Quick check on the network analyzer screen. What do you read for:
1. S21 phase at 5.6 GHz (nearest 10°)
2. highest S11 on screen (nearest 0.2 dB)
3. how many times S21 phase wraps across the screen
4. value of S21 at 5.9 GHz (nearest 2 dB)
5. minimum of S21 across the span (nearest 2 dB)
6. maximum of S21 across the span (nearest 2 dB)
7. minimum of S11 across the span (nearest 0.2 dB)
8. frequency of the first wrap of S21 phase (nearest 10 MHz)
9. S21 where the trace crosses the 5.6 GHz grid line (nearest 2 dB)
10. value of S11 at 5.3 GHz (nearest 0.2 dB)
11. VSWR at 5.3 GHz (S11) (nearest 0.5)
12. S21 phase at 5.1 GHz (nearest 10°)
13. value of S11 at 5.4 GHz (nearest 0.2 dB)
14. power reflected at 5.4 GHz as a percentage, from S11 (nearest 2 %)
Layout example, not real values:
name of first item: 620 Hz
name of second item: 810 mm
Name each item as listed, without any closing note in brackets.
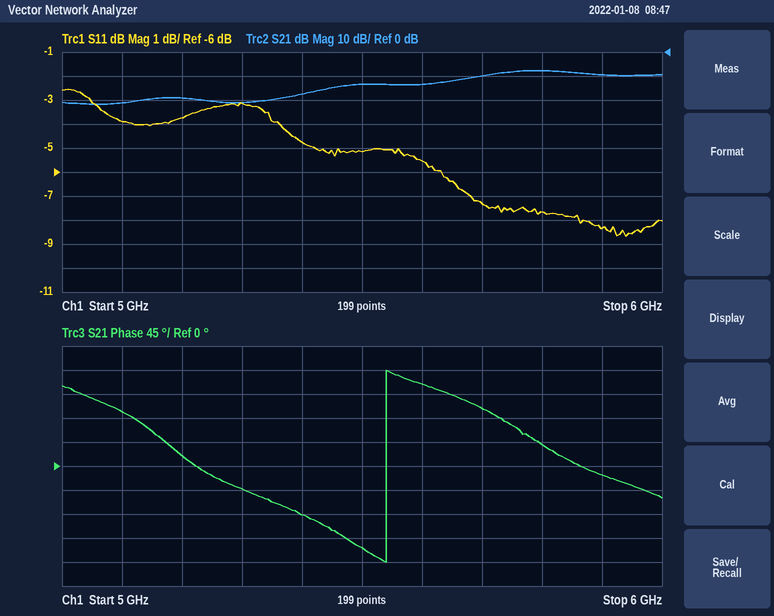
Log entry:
S21 phase at 5.6 GHz: 150°
highest S11 on screen: -2.6 dB
how many times S21 phase wraps across the screen: 1
value of S21 at 5.9 GHz: -10 dB
minimum of S21 across the span: -22 dB
maximum of S21 across the span: -8 dB
minimum of S11 across the span: -8.6 dB
frequency of the first wrap of S21 phase: 5.54 GHz
S21 where the trace crosses the 5.6 GHz grid line: -14 dB
value of S11 at 5.3 GHz: -3.2 dB
VSWR at 5.3 GHz (S11): 5.5
S21 phase at 5.1 GHz: 100°
value of S11 at 5.4 GHz: -4.8 dB
power reflected at 5.4 GHz as a percentage, from S11: 34 %
